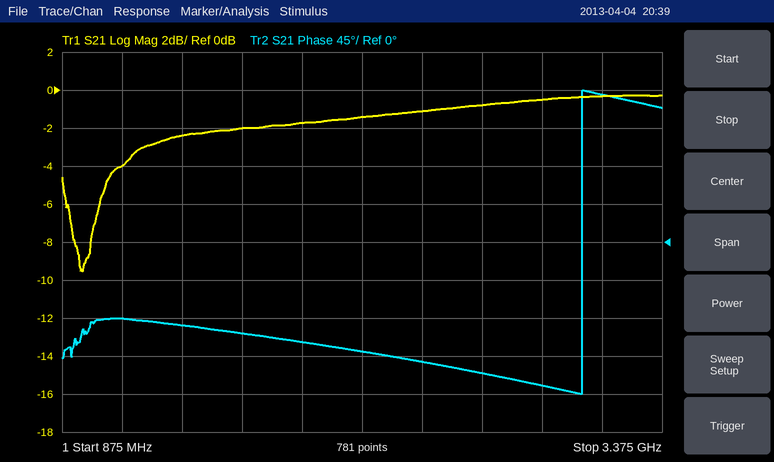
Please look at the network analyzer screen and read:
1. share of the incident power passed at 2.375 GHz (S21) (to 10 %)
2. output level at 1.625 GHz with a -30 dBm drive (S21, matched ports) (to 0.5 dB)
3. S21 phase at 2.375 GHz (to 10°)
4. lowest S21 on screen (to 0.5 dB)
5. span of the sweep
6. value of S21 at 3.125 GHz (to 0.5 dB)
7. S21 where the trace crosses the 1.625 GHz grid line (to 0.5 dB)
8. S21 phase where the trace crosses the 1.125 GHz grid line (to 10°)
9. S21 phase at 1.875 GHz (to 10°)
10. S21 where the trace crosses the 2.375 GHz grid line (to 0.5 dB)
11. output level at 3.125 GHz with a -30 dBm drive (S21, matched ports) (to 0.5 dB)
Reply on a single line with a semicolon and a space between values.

80 %; -32.0 dBm; -140°; -9.5 dB; 2.5 GHz; -0.5 dB; -2.0 dB; -90°; -120°; -1.0 dB; -30.5 dBm
